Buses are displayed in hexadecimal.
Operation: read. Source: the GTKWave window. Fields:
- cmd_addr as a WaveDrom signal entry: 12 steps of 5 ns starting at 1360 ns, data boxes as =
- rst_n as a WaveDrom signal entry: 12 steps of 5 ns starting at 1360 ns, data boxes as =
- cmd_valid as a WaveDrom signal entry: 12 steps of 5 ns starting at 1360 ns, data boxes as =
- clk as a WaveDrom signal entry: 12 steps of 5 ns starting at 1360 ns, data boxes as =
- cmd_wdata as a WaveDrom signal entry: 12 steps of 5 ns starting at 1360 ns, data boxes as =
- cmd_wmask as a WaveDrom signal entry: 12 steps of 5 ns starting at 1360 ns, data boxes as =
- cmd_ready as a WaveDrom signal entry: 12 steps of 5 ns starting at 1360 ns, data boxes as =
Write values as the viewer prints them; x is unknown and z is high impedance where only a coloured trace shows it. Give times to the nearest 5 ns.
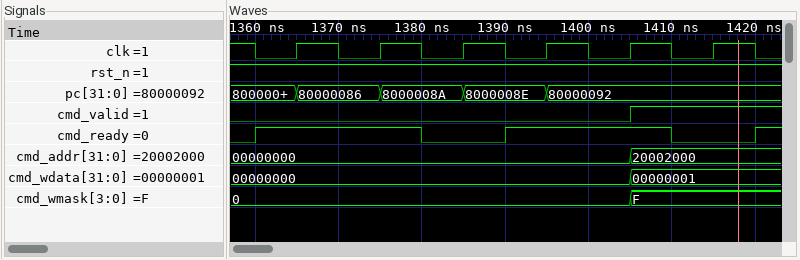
{name: 'cmd_addr', wave: '=........=..', data: '00000000 20002000'}
{name: 'rst_n', wave: '1...........'}
{name: 'cmd_valid', wave: '0........1..'}
{name: 'clk', wave: '010101010101'}
{name: 'cmd_wdata', wave: '=........=..', data: '00000000 00000001'}
{name: 'cmd_wmask', wave: '=........=..', data: '0 F'}
{name: 'cmd_ready', wave: '1...0.1...0.'}
